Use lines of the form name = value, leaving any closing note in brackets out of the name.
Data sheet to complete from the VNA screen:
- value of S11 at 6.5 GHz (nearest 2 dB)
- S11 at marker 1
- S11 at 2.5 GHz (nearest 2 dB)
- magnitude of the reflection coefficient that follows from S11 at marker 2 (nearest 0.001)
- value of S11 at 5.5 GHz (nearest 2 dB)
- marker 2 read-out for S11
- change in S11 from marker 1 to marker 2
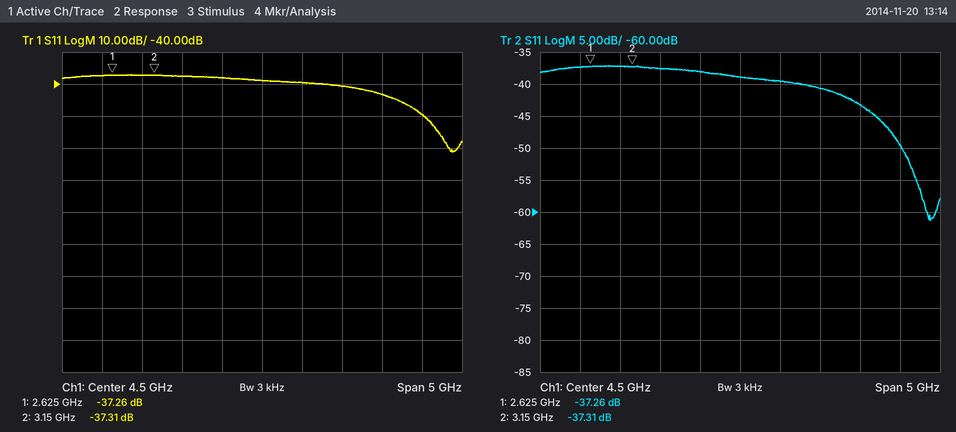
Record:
value of S11 at 6.5 GHz = -50 dB
S11 at marker 1 = -37.26 dB
S11 at 2.5 GHz = -38 dB
magnitude of the reflection coefficient that follows from S11 at marker 2 = 0.014
value of S11 at 5.5 GHz = -40 dB
marker 2 read-out for S11 = -37.31 dB
change in S11 from marker 1 to marker 2 = -0.05 dB
